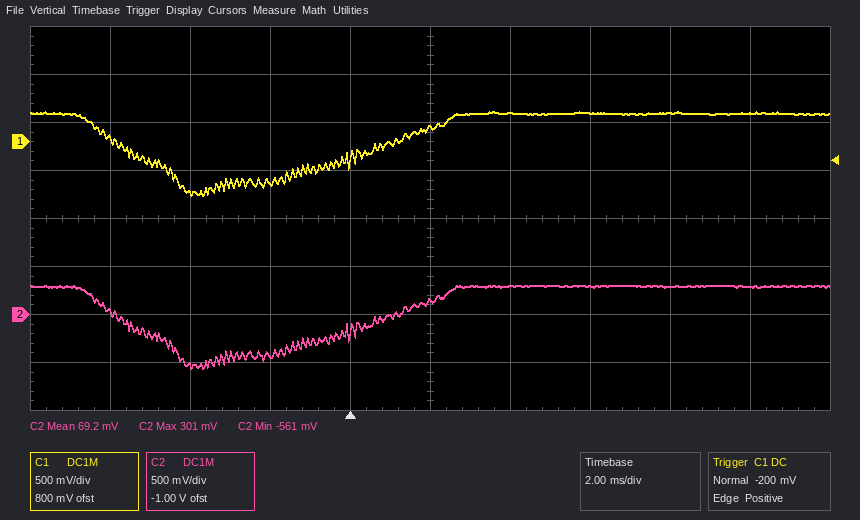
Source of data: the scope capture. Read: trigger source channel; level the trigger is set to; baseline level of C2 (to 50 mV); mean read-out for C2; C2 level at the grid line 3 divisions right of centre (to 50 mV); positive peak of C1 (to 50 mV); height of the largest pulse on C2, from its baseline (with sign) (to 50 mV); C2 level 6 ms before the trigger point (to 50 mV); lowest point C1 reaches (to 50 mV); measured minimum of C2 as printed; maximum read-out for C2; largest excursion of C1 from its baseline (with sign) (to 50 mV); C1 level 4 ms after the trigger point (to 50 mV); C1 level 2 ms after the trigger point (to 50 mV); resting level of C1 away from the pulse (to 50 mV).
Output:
C1
-200 mV
300 mV
69.2 mV
300 mV
300 mV
-850 mV
0 mV
-550 mV
-561 mV
301 mV
-850 mV
300 mV
150 mV
300 mV
